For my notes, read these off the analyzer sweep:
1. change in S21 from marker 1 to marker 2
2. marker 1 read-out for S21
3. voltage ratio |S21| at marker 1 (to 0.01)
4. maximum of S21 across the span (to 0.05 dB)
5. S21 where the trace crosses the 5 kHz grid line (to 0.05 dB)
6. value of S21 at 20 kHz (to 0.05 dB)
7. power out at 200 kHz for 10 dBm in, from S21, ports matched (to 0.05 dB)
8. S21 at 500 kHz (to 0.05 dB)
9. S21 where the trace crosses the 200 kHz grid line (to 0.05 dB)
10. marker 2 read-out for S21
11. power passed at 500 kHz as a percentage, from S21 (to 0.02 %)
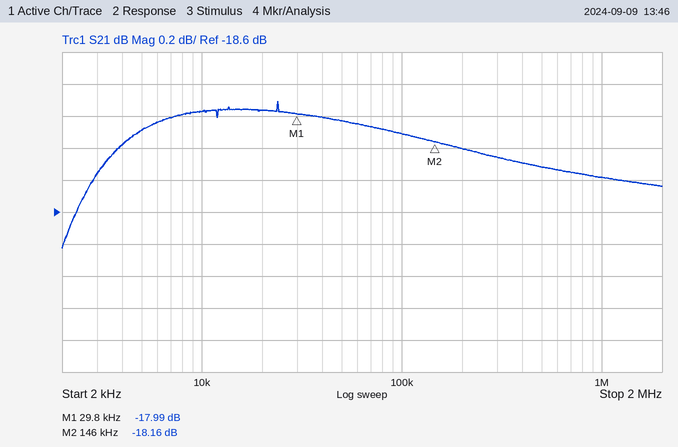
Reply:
-0.17 dB
-17.99 dB
0.13
-17.90 dB
-18.10 dB
-17.95 dB
-8.20 dBm
-18.30 dB
-18.20 dB
-18.16 dB
1.48 %
